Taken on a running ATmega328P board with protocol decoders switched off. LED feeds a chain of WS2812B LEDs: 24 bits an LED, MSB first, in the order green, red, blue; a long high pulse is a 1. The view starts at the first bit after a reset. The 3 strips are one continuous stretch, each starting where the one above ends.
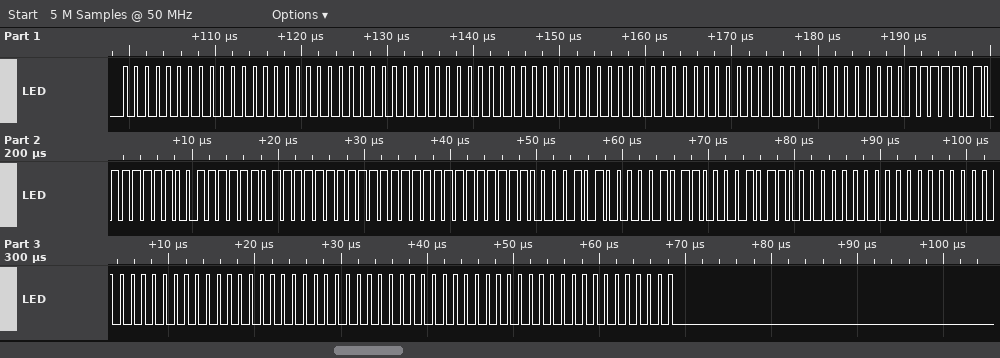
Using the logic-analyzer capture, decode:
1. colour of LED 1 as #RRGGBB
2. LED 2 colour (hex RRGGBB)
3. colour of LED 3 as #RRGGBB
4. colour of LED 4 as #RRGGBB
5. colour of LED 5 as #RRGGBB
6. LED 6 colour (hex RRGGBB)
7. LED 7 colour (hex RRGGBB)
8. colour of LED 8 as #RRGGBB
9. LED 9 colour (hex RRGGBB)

#000000
#000000
#000000
#7E7D7E
#FFFFFF
#0B0A0B
#000000
#000000
#000000
